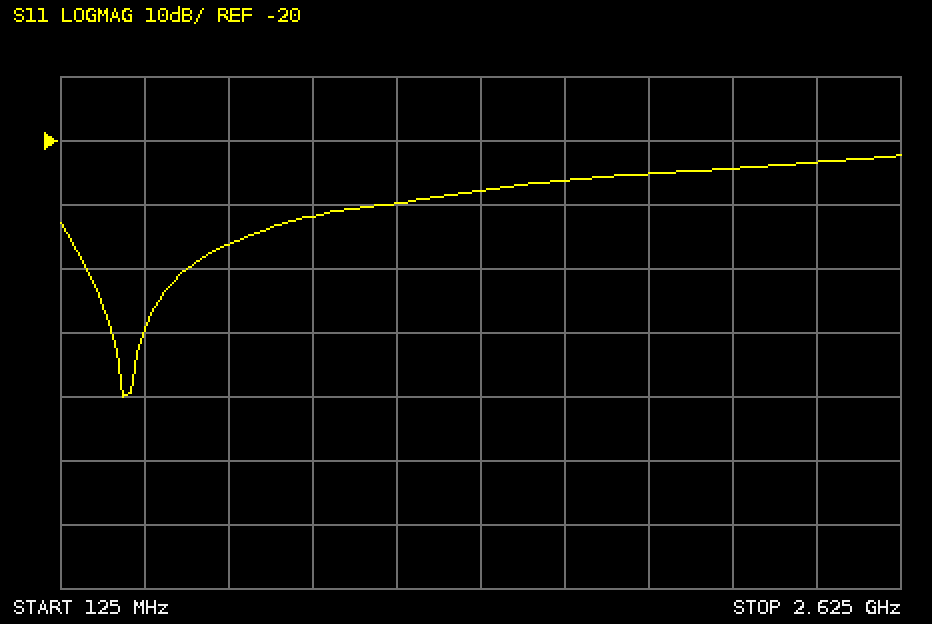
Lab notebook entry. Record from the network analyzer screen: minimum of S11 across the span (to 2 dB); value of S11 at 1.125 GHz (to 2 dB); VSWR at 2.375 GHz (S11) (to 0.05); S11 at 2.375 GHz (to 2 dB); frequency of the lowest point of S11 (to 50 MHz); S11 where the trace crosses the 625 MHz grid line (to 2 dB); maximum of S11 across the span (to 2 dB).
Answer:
-60 dB
-30 dB
1.15
-24 dB
300 MHz
-36 dB
-22 dB
